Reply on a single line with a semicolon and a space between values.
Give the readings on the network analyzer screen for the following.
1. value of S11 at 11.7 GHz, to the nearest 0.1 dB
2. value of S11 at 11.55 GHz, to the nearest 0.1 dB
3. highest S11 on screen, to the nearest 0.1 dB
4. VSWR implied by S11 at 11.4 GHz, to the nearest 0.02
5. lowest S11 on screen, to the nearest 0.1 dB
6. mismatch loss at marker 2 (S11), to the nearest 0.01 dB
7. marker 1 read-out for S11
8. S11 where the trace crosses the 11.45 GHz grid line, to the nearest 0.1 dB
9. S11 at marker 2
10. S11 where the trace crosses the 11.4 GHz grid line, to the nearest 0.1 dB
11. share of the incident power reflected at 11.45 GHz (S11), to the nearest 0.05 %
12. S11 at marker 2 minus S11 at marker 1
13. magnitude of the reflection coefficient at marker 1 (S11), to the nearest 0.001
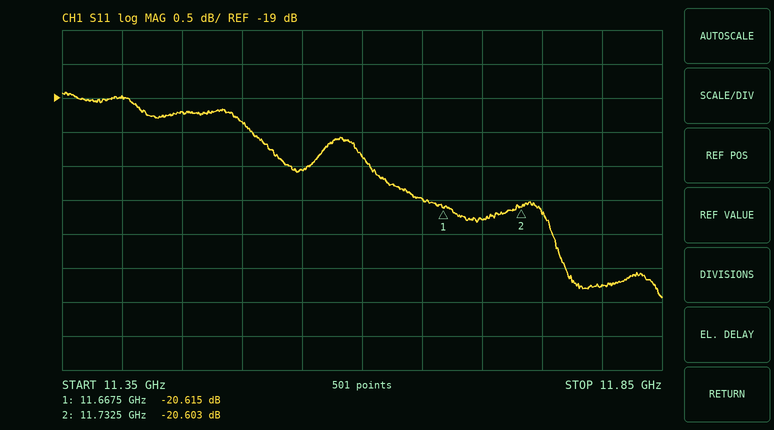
-20.8 dB; -20.1 dB; -18.9 dB; 1.26; -21.9 dB; 0.04 dB; -20.615 dB; -19.2 dB; -20.603 dB; -19.0 dB; 1.20 %; 0.012 dB; 0.093
